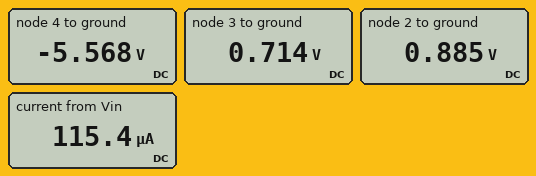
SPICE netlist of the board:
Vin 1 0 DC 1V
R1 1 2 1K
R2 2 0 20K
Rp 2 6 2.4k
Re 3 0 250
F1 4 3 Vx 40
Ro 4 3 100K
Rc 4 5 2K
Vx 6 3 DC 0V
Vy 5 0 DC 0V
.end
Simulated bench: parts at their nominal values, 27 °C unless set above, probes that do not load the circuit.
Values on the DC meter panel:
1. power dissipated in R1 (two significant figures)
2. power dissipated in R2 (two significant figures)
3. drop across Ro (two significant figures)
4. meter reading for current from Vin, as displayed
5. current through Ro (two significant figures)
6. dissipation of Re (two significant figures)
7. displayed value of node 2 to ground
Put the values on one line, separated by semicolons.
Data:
13 µW; 39 µW; 6.3 V; 115.4 µA; 63 µA; 2.0 mW; 0.885 V
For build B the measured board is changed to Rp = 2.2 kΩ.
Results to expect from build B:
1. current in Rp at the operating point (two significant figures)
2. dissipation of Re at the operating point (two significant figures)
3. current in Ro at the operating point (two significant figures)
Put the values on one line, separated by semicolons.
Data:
72 µA; 2.1 mW; 64 µA
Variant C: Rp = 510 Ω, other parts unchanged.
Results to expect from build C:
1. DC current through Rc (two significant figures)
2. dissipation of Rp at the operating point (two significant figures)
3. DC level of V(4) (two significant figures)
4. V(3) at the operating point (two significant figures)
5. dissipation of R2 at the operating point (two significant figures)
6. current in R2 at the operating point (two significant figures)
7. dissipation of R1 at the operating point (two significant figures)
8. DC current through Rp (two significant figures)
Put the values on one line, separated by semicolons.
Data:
3.2 mA; 3.5 µW; -6.5 V; 830 mV; 38 µW; 44 µA; 16 µW; 83 µA
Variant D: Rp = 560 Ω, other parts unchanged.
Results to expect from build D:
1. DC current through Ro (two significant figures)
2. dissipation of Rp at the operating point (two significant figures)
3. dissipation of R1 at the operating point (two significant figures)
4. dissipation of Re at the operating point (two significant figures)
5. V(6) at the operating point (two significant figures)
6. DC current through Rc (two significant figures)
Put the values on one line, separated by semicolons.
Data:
73 µA; 3.8 µW; 16 µW; 2.7 mW; 830 mV; 3.2 mA
